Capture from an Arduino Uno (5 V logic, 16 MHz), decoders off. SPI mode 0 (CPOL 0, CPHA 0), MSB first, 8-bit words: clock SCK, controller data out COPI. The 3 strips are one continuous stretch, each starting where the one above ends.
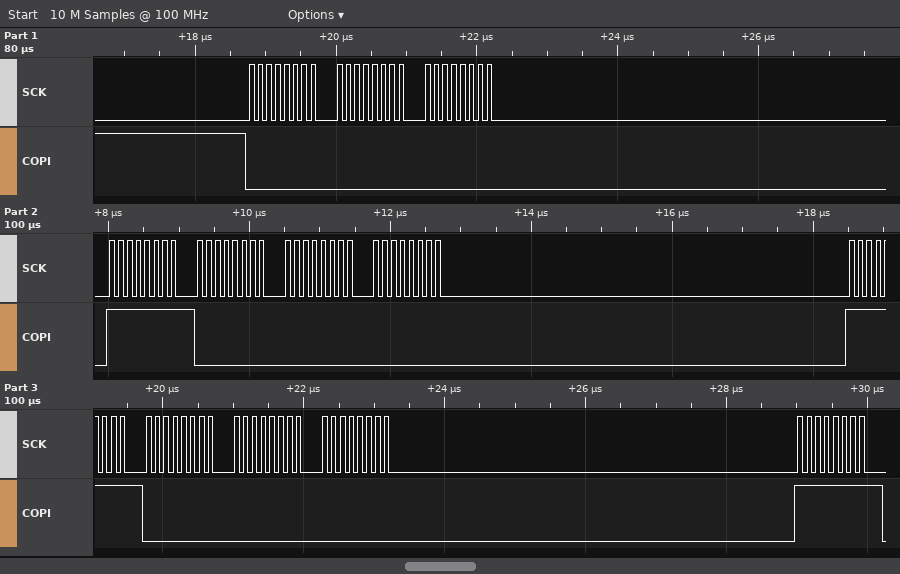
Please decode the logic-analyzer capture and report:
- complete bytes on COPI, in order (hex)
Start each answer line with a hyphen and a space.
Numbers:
- 0x00 0x00 0x00 0xFF 0x00 0x00 0x00 0xFF 0x00 0x00 0x00 0xFF
